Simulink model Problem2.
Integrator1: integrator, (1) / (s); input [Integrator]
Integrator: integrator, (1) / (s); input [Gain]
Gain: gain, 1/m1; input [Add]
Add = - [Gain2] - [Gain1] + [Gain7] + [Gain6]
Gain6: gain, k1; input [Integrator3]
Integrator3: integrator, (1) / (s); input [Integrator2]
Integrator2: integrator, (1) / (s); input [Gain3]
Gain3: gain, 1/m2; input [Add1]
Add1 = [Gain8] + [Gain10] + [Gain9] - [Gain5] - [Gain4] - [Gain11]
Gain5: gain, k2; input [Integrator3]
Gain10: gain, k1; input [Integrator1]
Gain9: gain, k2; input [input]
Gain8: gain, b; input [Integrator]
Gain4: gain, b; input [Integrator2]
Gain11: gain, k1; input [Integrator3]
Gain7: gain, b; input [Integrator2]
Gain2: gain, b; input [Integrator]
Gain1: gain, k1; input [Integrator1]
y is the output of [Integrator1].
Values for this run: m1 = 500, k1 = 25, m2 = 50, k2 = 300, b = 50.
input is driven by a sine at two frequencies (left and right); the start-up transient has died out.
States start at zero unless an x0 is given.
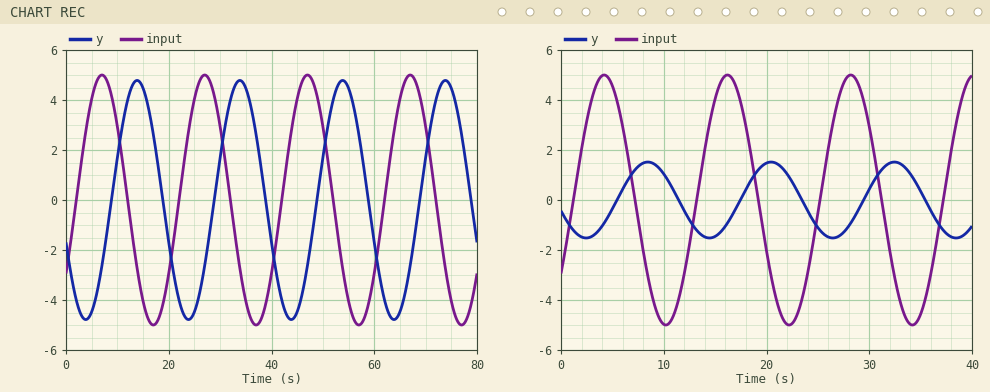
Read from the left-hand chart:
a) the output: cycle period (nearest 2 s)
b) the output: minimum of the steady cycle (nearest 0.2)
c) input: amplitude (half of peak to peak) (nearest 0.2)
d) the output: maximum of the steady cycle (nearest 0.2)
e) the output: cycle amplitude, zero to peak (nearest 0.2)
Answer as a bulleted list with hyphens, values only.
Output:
- 20 s
- -4.8
- 5.0
- 4.8
- 4.8
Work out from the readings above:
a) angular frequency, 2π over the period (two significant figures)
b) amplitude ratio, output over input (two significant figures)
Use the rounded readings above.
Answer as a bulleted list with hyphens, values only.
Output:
- 0.31 rad/s
- 0.96
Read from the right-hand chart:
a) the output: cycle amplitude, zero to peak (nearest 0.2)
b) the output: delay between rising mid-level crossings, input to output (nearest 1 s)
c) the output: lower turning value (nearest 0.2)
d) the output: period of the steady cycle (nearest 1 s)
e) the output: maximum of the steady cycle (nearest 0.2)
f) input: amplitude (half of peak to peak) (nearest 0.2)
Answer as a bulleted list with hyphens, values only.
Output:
- 1.6
- 4 s
- -1.6
- 12 s
- 1.6
- 5.0
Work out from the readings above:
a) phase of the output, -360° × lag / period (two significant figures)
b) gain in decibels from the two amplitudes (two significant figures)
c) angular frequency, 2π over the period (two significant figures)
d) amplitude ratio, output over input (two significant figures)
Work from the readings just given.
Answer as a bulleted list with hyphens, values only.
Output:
- -120°
- -9.9 dB
- 0.52 rad/s
- 0.32
